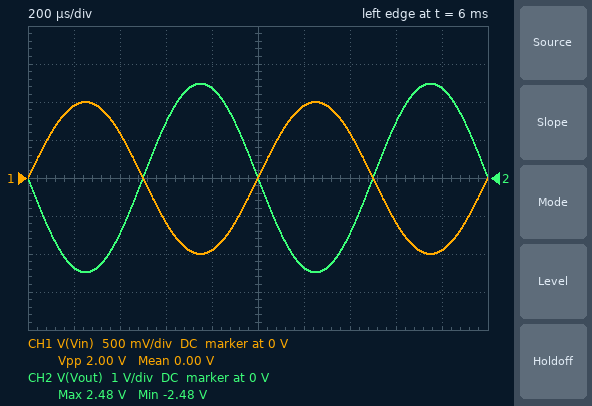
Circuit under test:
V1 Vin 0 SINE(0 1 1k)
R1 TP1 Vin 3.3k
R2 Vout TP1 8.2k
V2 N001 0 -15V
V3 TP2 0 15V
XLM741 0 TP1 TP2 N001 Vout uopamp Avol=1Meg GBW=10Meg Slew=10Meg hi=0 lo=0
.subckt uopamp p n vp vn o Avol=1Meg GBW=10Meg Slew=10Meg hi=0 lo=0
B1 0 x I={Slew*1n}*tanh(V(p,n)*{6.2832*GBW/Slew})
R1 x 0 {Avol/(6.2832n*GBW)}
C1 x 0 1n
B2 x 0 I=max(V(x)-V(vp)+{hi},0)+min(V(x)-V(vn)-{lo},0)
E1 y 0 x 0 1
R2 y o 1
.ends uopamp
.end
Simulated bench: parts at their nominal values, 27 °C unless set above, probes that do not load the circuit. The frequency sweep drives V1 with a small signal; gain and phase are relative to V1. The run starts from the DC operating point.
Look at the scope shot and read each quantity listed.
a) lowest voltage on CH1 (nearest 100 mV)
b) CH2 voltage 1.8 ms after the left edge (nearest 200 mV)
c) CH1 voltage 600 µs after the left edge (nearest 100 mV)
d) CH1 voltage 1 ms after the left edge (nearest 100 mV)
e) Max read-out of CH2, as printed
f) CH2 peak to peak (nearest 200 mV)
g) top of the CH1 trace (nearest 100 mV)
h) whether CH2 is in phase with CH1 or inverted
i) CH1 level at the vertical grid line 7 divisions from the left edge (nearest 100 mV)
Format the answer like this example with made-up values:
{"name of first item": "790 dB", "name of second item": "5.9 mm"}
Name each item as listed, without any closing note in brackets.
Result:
{"lowest voltage on CH1": "-1.0 V", "CH2 voltage 1.8 ms after the left edge": "2.4 V", "CH1 voltage 600 µs after the left edge": "-600 mV", "CH1 voltage 1 ms after the left edge": "0 V", "Max read-out of CH2, as printed": "2.48 V", "CH2 peak to peak": "5.0 V", "top of the CH1 trace": "1.0 V", "whether CH2 is in phase with CH1 or inverted": "inverted", "CH1 level at the vertical grid line 7 divisions from the left edge": "600 mV"}
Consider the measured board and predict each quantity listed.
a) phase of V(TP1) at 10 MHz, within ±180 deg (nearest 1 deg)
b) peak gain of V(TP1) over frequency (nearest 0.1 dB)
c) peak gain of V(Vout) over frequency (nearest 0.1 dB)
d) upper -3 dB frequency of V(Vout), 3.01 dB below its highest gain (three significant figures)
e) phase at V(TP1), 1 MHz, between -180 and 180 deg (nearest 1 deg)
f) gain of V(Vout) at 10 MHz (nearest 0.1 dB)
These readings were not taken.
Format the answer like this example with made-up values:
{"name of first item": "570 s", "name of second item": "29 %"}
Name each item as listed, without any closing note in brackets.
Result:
{"phase of V(TP1) at 10 MHz, within ±180 deg": "16 deg", "peak gain of V(TP1) over frequency": "-2.9 dB", "peak gain of V(Vout) over frequency": "7.9 dB", "upper -3 dB frequency of V(Vout), 3.01 dB below its highest gain": "2.87 MHz", "phase at V(TP1), 1 MHz, between -180 and 180 deg": "71 deg", "gain of V(Vout) at 10 MHz": "-3.3 dB"}
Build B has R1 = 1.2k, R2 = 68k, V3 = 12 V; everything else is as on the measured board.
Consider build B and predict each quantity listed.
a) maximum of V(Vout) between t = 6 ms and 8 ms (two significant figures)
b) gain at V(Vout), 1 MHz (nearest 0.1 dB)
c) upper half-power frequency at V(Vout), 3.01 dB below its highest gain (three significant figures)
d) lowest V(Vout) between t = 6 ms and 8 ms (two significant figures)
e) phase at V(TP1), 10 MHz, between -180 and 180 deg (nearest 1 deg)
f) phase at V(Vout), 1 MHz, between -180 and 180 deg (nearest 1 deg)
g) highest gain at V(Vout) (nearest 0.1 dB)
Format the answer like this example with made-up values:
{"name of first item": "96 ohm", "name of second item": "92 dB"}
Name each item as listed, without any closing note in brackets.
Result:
{"maximum of V(Vout) between t = 6 ms and 8 ms": "12 V", "gain at V(Vout), 1 MHz": "19.7 dB", "upper half-power frequency at V(Vout), 3.01 dB below its highest gain": "173 kHz", "lowest V(Vout) between t = 6 ms and 8 ms": "-15 V", "phase at V(TP1), 10 MHz, between -180 and 180 deg": "1 deg", "phase at V(Vout), 1 MHz, between -180 and 180 deg": "100 deg", "highest gain at V(Vout)": "35.1 dB"}
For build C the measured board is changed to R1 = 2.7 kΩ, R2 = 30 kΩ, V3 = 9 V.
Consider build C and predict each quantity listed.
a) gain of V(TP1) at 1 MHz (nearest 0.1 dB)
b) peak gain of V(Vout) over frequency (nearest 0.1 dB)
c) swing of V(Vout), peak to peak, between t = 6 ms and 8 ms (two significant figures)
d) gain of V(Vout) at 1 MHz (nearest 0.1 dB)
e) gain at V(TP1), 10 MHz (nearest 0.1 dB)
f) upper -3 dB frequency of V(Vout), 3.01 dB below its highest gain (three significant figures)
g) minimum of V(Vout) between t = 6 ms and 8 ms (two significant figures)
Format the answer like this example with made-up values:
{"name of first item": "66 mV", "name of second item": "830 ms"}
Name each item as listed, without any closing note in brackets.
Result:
{"gain of V(TP1) at 1 MHz": "-3.0 dB", "peak gain of V(Vout) over frequency": "20.9 dB", "swing of V(Vout), peak to peak, between t = 6 ms and 8 ms": "20 V", "gain of V(Vout) at 1 MHz": "17.0 dB", "gain at V(TP1), 10 MHz": "-0.8 dB", "upper -3 dB frequency of V(Vout), 3.01 dB below its highest gain": "826 kHz", "minimum of V(Vout) between t = 6 ms and 8 ms": "-11 V"}
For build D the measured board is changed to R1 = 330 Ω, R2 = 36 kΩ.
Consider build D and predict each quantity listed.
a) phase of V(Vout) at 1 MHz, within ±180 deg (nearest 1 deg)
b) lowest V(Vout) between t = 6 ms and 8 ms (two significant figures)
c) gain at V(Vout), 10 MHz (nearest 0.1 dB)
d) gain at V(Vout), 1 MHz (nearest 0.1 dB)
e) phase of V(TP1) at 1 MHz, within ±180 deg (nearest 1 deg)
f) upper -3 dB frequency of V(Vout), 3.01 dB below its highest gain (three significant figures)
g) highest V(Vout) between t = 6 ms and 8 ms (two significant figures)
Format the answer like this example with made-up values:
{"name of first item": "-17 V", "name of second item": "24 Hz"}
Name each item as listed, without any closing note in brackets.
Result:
{"phase of V(Vout) at 1 MHz, within ±180 deg": "95 deg", "lowest V(Vout) between t = 6 ms and 8 ms": "-15 V", "gain at V(Vout), 10 MHz": "-0.1 dB", "gain at V(Vout), 1 MHz": "19.9 dB", "phase of V(TP1) at 1 MHz, within ±180 deg": "5 deg", "upper -3 dB frequency of V(Vout), 3.01 dB below its highest gain": "90.8 kHz", "highest V(Vout) between t = 6 ms and 8 ms": "15 V"}
